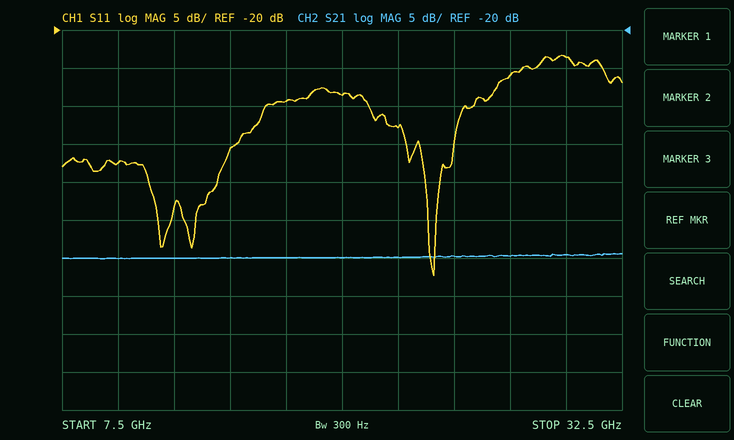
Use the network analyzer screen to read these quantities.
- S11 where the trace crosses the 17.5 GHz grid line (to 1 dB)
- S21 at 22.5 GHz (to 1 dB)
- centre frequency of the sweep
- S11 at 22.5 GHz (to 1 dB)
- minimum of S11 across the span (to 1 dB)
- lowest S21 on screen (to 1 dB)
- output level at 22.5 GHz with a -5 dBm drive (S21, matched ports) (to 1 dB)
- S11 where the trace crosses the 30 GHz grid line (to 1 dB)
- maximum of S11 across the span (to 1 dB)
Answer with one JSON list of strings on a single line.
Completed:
["-29 dB", "-50 dB", "20 GHz", "-33 dB", "-52 dB", "-50 dB", "-55 dBm", "-24 dB", "-23 dB"]
